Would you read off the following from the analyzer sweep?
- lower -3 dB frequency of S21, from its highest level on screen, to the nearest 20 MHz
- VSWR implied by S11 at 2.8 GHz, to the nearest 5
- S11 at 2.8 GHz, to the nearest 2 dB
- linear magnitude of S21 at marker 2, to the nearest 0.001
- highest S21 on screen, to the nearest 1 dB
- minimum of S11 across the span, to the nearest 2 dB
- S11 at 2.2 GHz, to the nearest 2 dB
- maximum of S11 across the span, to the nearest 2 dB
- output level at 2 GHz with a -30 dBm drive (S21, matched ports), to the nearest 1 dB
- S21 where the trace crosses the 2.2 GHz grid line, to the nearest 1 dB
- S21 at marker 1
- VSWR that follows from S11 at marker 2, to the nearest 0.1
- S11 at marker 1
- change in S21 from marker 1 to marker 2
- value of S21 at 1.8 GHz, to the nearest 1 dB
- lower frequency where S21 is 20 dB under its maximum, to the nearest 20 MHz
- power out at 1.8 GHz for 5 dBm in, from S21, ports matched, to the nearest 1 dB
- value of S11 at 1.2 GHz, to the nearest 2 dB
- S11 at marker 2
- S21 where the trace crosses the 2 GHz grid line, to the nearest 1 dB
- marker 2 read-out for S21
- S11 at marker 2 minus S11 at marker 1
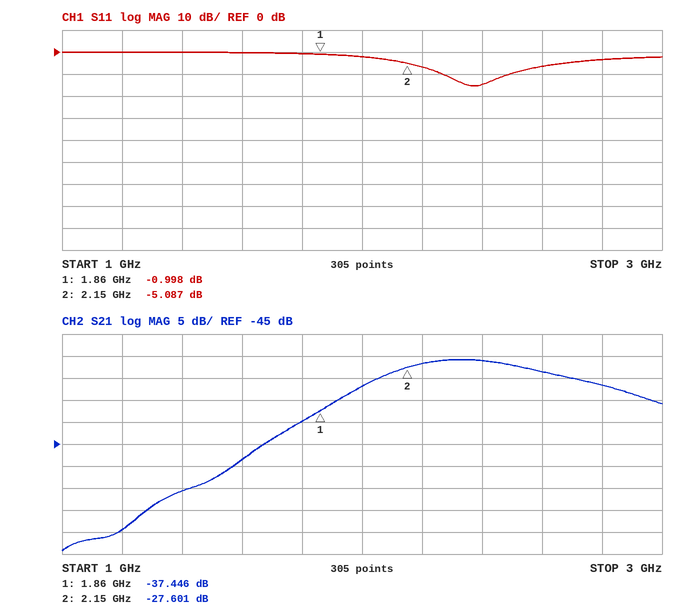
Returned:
2.10 GHz
5
-4 dB
0.042
-26 dB
-16 dB
-6 dB
0 dB
-62 dBm
-27 dB
-37.446 dB
3.5
-0.998 dB
9.845 dB
-40 dB
1.66 GHz
-35 dBm
0 dB
-5.087 dB
-32 dB
-27.601 dB
-4.089 dB
